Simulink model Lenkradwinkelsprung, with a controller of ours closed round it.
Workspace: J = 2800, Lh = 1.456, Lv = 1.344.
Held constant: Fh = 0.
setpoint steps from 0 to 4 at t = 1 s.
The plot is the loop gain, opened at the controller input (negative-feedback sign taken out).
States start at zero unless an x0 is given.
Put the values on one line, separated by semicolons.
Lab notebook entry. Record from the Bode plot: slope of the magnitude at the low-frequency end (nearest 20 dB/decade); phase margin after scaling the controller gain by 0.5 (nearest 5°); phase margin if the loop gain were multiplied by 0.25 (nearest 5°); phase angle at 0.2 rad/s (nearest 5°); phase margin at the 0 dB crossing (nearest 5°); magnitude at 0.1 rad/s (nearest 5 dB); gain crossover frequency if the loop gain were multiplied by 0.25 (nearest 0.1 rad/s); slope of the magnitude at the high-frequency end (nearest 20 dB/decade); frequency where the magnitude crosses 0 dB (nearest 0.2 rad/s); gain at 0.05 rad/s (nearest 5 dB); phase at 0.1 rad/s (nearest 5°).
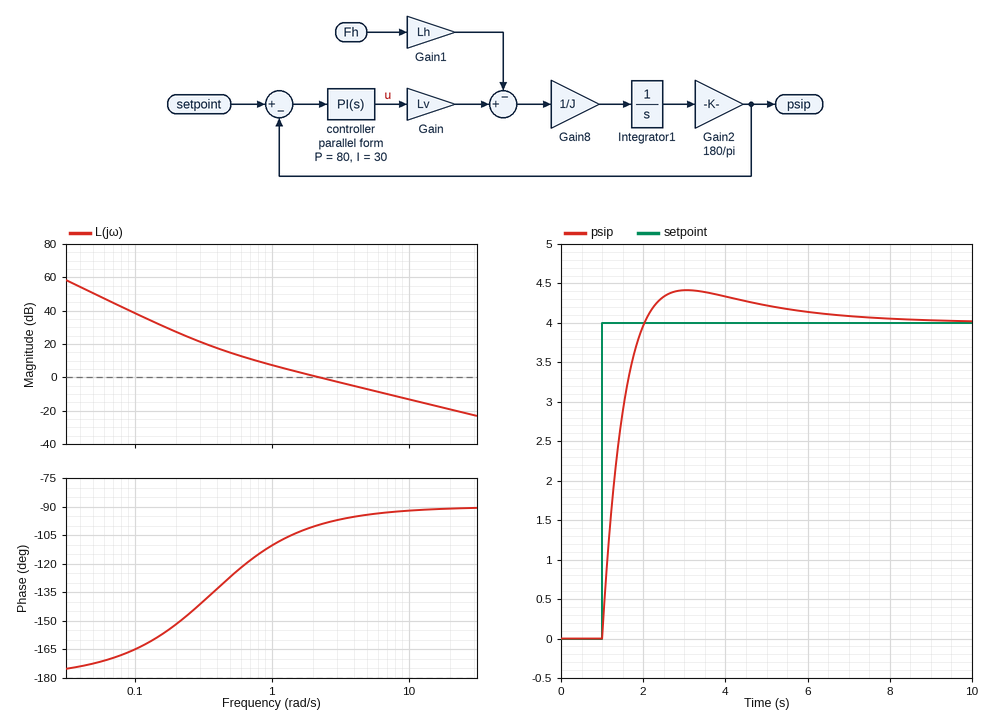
-40 dB/decade; 70°; 60°; -150°; 80°; 40 dB; 0.6 rad/s; -20 dB/decade; 2.2 rad/s; 50 dB; -165°
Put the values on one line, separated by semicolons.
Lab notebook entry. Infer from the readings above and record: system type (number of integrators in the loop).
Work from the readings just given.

2
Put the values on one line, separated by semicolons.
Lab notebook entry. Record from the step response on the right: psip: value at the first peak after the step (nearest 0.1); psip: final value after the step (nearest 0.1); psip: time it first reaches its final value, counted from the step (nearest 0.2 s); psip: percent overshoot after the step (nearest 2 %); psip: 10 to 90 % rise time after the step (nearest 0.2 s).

4.4; 4.0; 1.0 s; 10 %; 0.8 s
